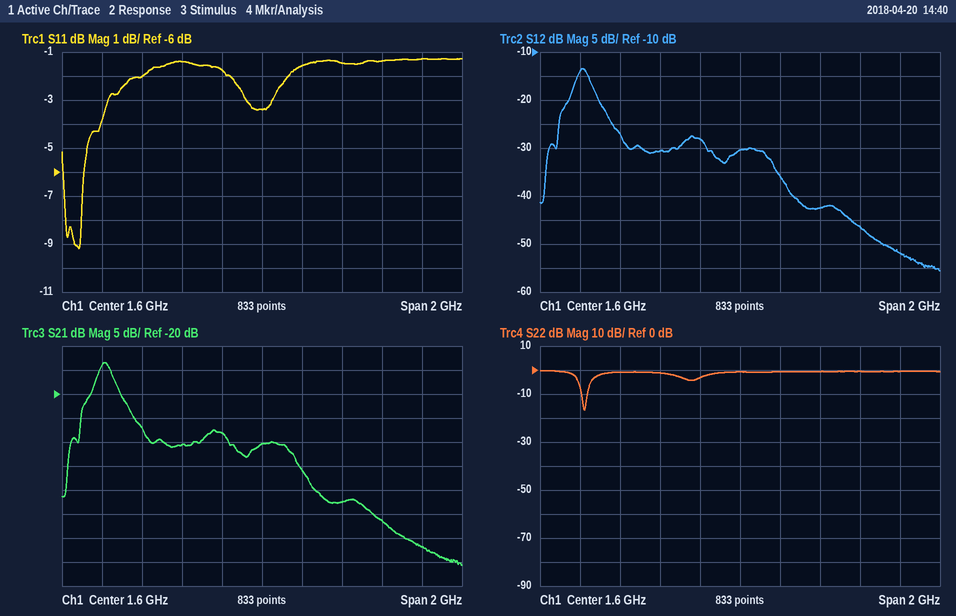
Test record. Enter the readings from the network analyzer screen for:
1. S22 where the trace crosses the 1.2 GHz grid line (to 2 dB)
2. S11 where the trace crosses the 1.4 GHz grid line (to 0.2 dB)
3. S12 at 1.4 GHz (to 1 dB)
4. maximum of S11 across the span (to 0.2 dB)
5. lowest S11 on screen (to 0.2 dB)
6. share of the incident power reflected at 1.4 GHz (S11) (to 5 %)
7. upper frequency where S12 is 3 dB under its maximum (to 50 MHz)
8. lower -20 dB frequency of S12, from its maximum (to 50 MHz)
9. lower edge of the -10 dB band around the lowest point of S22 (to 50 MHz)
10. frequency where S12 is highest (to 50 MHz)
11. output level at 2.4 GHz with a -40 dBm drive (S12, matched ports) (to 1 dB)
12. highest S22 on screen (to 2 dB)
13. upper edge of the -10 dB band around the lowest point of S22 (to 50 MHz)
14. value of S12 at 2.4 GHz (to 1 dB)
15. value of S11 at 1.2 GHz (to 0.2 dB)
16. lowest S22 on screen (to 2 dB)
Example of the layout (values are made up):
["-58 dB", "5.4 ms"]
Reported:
["-2 dB", "-1.8 dB", "-28 dB", "-1.2 dB", "-9.2 dB", "65 %", "850 MHz", "650 MHz", "800 MHz", "800 MHz", "-92 dBm", "0 dB", "850 MHz", "-52 dB", "-1.4 dB", "-16 dB"]
